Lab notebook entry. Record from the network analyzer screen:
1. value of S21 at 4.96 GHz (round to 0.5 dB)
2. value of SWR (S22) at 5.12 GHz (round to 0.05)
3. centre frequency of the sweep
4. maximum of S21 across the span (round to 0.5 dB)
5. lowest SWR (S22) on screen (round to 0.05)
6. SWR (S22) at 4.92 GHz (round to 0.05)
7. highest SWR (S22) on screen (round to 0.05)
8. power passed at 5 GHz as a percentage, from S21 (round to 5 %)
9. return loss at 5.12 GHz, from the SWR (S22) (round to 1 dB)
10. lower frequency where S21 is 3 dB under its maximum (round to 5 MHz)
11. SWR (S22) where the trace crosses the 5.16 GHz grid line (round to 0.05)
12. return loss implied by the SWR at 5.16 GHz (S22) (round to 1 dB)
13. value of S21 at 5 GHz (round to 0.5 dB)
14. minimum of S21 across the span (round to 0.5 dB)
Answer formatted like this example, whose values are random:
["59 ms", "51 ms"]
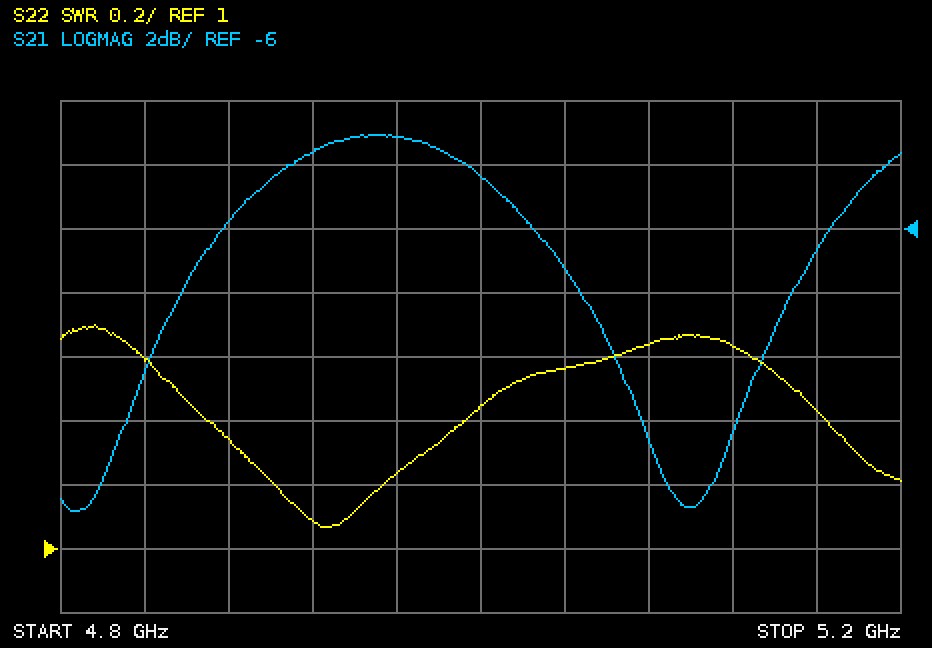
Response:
["-3.0 dB", "1.65", "5 GHz", "-3.0 dB", "1.05", "1.10", "1.70", "35 %", "12 dB", "4.875 GHz", "1.45", "15 dB", "-4.5 dB", "-15.0 dB"]
